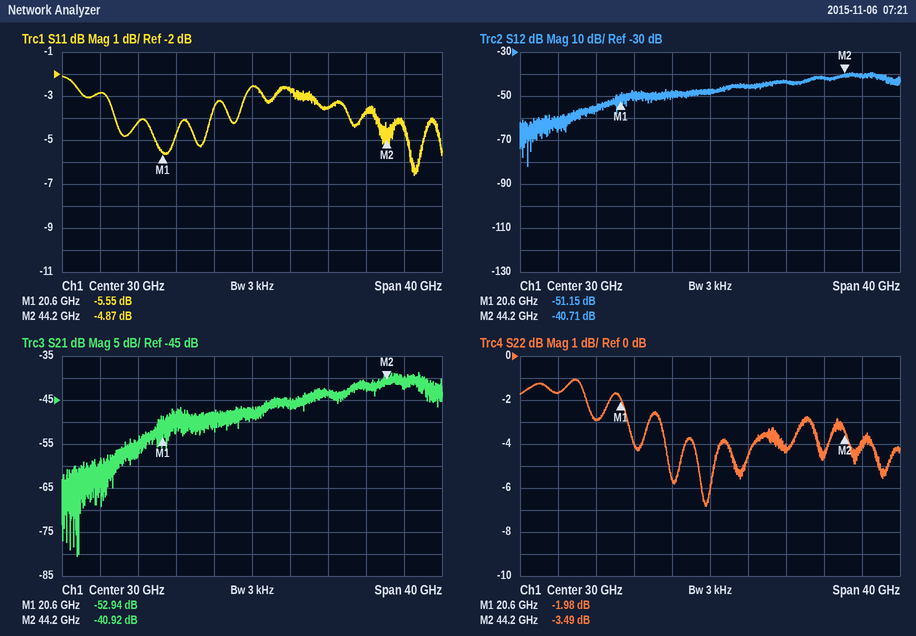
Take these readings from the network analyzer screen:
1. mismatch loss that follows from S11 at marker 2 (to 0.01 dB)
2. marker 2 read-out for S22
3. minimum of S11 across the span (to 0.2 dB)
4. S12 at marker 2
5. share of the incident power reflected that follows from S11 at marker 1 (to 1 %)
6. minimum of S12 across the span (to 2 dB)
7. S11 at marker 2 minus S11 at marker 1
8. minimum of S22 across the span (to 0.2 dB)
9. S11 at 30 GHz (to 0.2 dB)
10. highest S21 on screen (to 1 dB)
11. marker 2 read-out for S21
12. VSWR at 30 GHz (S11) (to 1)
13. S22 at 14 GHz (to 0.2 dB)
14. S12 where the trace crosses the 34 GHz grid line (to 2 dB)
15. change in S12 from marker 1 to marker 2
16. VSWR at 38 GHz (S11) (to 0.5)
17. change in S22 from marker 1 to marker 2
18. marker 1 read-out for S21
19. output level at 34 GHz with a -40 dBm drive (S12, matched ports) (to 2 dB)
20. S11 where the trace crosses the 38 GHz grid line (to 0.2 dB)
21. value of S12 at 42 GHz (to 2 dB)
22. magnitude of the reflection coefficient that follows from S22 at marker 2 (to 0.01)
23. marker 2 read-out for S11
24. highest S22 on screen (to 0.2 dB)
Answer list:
1.71 dB
-3.49 dB
-6.6 dB
-40.71 dB
28 %
-82 dB
0.68 dB
-6.8 dB
-2.6 dB
-39 dB
-40.92 dB
7
-1.6 dB
-46 dB
10.44 dB
5.0
-1.51 dB
-52.94 dB
-86 dBm
-3.6 dB
-42 dB
0.67
-4.87 dB
-1.0 dB
